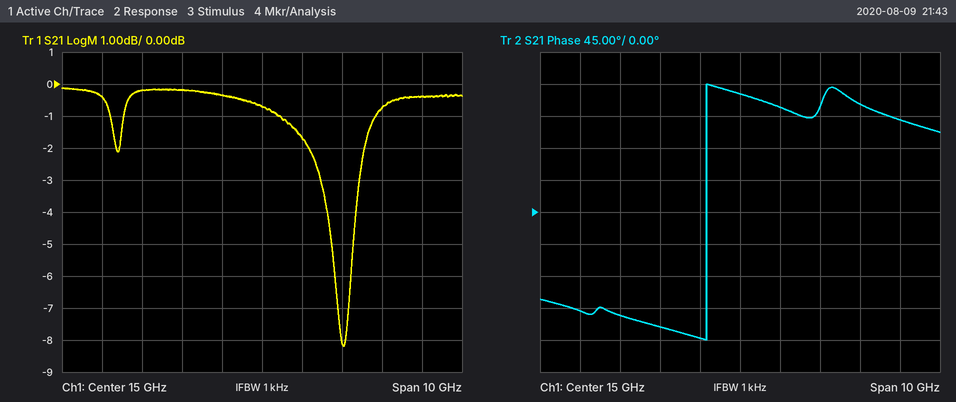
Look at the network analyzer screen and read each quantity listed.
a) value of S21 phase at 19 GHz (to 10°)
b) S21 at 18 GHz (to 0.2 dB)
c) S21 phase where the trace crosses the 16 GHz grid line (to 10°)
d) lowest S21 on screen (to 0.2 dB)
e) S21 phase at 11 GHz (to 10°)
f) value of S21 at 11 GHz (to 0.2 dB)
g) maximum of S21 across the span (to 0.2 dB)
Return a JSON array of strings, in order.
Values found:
["130°", "-0.8 dB", "150°", "-8.2 dB", "-140°", "-0.4 dB", "-0.2 dB"]
